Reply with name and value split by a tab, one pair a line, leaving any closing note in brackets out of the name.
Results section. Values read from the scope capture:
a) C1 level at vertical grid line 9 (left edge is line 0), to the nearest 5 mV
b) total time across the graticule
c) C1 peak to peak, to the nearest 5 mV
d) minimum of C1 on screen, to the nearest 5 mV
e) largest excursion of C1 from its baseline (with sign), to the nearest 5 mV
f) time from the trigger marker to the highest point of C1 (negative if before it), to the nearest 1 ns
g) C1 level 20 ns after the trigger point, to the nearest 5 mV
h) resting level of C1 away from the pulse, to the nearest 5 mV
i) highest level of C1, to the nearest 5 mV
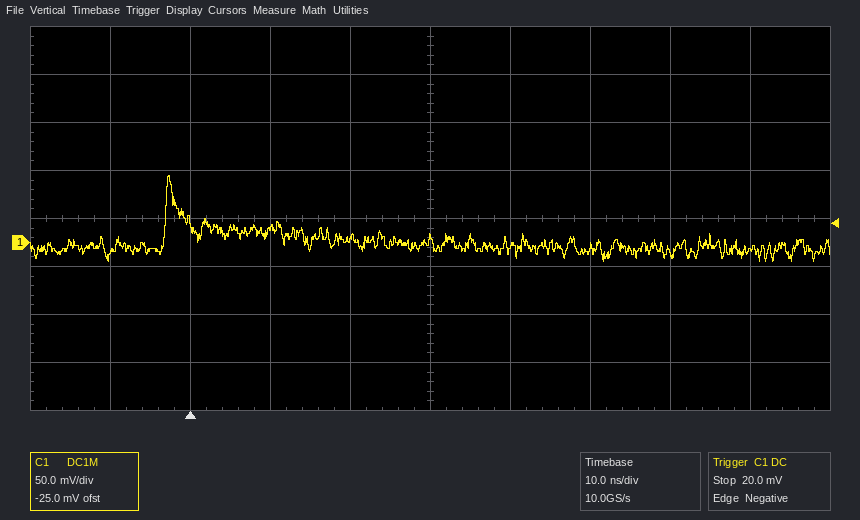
C1 level at vertical grid line 9 (left edge is line 0), to the nearest 5 mV	-10 mV
total time across the graticule	100 ns
C1 peak to peak, to the nearest 5 mV	90 mV
minimum of C1 on screen, to the nearest 5 mV	-20 mV
largest excursion of C1 from its baseline (with sign), to the nearest 5 mV	+75 mV
time from the trigger marker to the highest point of C1 (negative if before it), to the nearest 1 ns	-3 ns
C1 level 20 ns after the trigger point, to the nearest 5 mV	5 mV
resting level of C1 away from the pulse, to the nearest 5 mV	-5 mV
highest level of C1, to the nearest 5 mV	70 mV
